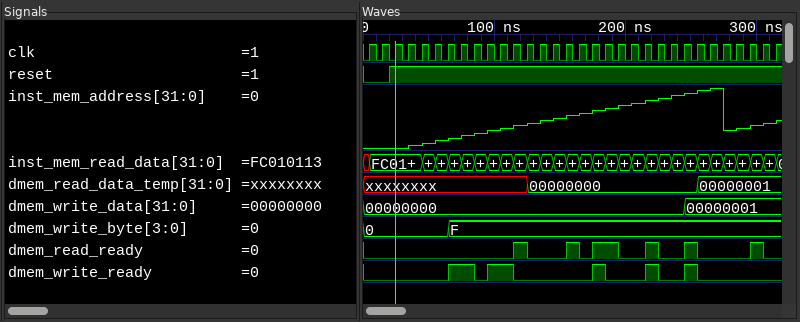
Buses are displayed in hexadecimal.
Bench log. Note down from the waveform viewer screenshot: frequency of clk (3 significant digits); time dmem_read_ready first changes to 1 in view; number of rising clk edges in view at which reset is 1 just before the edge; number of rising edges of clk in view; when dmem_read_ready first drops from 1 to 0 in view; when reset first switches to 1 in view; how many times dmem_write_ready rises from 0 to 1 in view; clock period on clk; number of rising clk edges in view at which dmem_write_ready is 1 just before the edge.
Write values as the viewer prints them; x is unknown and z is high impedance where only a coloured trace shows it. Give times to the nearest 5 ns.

100 MHz
115 ns
30
32
125 ns
20 ns
5
10 ns
7
